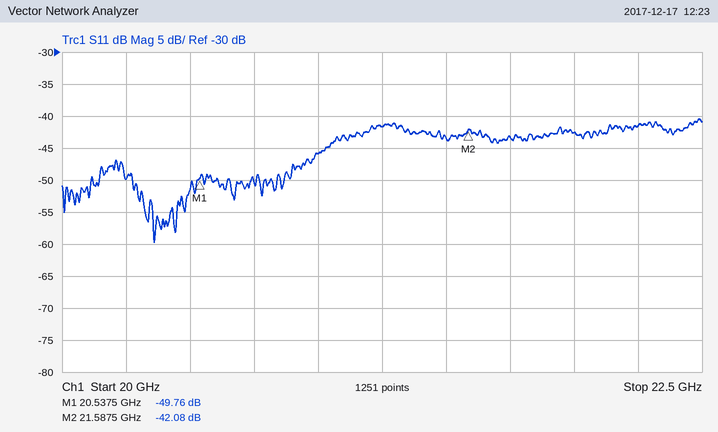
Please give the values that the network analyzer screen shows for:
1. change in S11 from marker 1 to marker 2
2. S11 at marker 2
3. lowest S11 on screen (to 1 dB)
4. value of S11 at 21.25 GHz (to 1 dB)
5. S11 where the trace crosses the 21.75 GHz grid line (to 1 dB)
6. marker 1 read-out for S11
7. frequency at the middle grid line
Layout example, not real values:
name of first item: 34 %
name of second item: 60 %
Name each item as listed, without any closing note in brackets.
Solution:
change in S11 from marker 1 to marker 2: 7.68 dB
S11 at marker 2: -42.08 dB
lowest S11 on screen: -60 dB
value of S11 at 21.25 GHz: -42 dB
S11 where the trace crosses the 21.75 GHz grid line: -43 dB
marker 1 read-out for S11: -49.76 dB
frequency at the middle grid line: 21.25 GHz
